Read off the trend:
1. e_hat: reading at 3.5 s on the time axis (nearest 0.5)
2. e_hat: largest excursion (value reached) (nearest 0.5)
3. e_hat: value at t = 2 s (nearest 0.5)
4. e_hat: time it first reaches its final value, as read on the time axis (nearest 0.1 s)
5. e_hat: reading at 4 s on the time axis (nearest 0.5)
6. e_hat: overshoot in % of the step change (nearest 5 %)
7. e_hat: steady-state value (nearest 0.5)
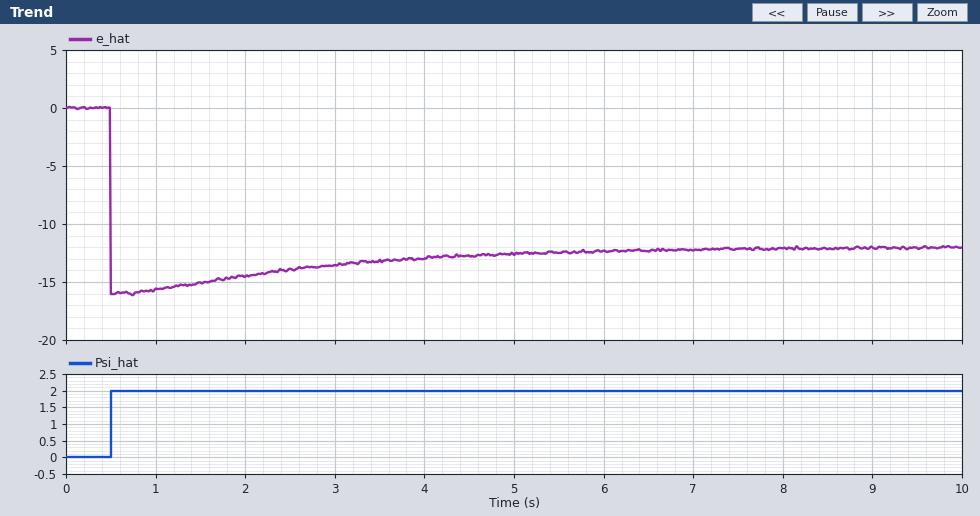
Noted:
-13.0
-16.0
-14.5
0.5 s
-13.0
35 %
-12.0
